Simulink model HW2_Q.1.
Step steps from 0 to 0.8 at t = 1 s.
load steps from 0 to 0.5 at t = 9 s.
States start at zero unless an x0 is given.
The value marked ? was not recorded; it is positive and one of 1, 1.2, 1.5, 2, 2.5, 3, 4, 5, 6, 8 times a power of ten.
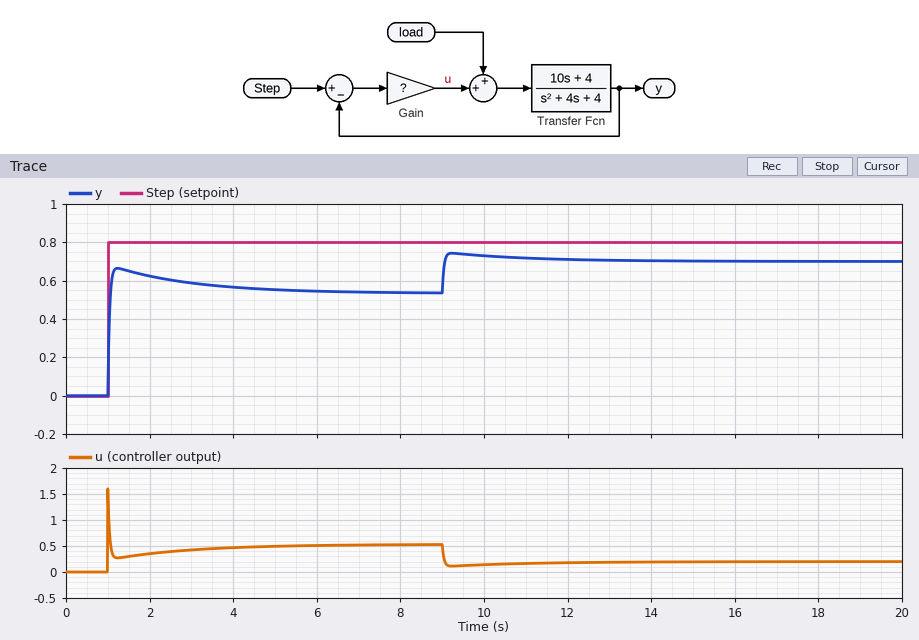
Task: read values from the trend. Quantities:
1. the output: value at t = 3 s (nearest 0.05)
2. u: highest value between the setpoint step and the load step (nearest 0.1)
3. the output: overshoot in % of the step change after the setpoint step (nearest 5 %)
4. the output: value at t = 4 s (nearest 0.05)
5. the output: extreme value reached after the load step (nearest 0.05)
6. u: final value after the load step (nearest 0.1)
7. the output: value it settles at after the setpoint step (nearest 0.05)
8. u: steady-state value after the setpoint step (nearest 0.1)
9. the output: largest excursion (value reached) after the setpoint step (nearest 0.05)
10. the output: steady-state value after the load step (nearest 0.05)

0.60
1.6
25 %
0.55
0.75
0.2
0.55
0.5
0.65
0.70
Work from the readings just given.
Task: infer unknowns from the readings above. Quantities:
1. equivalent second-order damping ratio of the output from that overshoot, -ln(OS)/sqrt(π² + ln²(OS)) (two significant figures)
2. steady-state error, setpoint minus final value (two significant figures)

0.40
0.25
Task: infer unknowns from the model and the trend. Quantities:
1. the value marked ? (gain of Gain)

2
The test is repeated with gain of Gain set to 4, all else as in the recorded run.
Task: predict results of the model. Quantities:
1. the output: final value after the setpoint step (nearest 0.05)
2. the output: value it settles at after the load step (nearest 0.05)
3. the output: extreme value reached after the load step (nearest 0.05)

0.65
0.75
0.75
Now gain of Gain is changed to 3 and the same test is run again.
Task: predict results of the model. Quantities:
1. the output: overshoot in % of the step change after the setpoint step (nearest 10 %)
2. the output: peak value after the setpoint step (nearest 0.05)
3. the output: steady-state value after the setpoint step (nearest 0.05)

20 %
0.70
0.60
